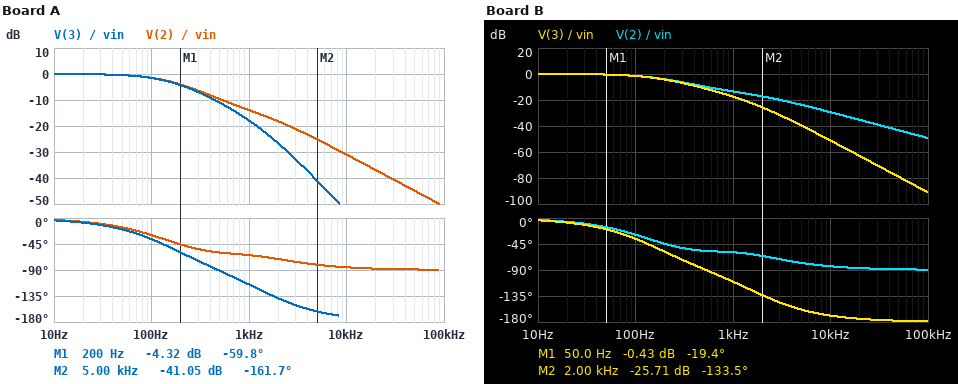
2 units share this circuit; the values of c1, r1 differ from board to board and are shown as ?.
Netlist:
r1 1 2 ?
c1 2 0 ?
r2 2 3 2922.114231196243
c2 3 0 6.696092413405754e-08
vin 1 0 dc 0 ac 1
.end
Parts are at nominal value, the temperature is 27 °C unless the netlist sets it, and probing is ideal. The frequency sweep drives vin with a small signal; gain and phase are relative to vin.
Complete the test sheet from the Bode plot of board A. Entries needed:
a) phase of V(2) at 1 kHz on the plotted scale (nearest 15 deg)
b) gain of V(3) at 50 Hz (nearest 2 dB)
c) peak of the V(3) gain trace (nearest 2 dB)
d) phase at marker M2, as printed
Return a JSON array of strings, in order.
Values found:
["-60 deg", "0 dB", "0 dB", "-161.7 deg"]
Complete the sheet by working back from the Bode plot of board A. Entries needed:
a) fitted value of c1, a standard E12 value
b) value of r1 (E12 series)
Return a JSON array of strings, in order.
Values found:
["100 nF", "5.6 kΩ"]
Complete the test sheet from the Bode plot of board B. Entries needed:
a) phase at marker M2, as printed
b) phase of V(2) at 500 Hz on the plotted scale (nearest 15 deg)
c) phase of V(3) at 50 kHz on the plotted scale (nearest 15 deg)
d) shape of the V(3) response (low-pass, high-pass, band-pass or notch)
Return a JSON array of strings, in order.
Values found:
["-133.5 deg", "-60 deg", "-180 deg", "low-pass"]
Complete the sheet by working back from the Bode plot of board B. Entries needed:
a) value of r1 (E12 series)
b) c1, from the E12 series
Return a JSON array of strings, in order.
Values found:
["6.8 kΩ", "68 nF"]
